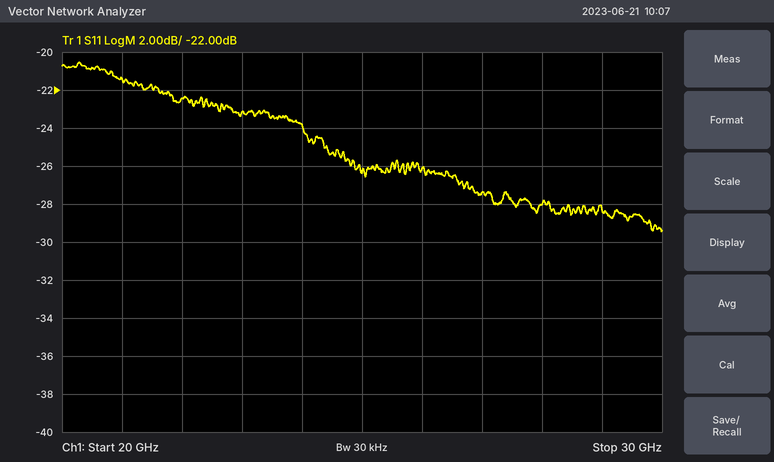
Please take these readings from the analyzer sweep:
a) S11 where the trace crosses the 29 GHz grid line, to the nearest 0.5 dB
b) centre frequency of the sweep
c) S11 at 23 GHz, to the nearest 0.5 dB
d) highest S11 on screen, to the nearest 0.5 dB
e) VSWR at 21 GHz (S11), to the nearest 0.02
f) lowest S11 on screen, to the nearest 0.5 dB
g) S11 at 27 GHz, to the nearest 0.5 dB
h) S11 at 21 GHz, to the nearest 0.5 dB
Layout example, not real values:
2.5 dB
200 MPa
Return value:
-28.5 dB
25 GHz
-23.0 dB
-20.5 dB
1.18
-29.5 dB
-27.5 dB
-21.5 dB
